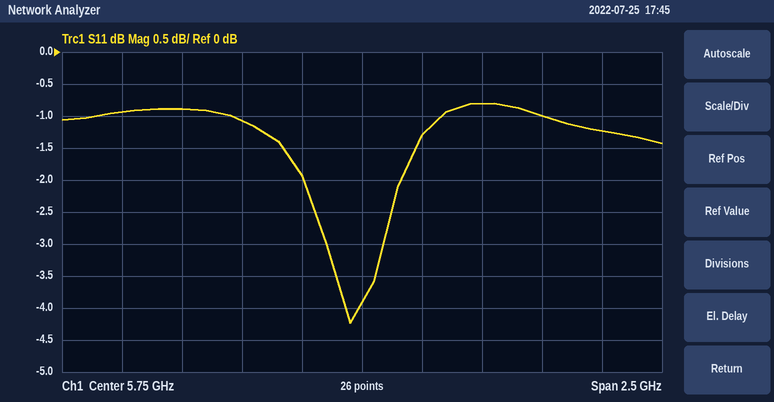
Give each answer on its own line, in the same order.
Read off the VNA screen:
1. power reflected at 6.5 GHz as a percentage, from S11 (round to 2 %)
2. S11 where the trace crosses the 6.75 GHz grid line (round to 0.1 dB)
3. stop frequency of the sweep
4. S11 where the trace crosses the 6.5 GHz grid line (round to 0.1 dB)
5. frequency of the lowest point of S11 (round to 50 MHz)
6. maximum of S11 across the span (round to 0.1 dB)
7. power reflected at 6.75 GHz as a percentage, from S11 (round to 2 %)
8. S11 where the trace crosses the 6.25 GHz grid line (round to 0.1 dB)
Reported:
80 %
-1.2 dB
7 GHz
-1.0 dB
5.70 GHz
-0.8 dB
76 %
-0.8 dB
